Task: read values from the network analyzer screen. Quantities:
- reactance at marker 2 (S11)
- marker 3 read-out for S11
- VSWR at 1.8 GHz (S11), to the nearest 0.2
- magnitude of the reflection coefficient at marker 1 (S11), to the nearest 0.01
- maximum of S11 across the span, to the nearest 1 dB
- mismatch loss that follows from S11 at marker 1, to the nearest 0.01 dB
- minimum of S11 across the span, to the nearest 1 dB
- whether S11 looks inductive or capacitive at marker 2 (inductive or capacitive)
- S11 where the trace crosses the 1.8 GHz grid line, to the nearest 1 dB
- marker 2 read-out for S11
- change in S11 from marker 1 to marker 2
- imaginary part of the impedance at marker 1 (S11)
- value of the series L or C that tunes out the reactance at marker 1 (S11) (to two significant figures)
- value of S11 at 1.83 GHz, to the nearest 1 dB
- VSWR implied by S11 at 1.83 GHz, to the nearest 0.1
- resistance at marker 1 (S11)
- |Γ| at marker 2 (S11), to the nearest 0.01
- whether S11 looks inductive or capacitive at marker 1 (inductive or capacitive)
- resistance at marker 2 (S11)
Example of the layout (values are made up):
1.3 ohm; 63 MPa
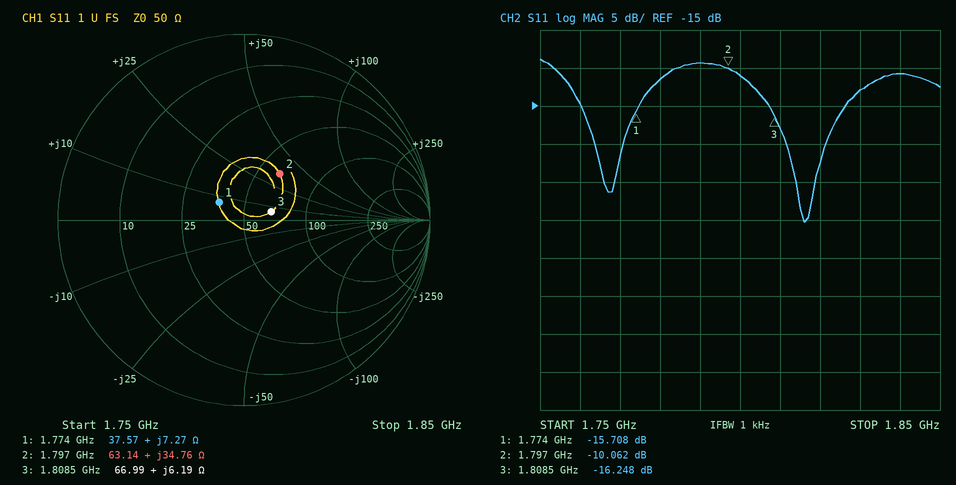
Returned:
+34.76 Ω; -16.248 dB; 1.8; 0.16; -9 dB; 0.12 dB; -30 dB; inductive; -11 dB; -10.062 dB; 5.646 dB; +7.27 Ω; 12 pF; -13 dB; 1.6; 37.57 Ω; 0.31; inductive; 63.14 Ω
